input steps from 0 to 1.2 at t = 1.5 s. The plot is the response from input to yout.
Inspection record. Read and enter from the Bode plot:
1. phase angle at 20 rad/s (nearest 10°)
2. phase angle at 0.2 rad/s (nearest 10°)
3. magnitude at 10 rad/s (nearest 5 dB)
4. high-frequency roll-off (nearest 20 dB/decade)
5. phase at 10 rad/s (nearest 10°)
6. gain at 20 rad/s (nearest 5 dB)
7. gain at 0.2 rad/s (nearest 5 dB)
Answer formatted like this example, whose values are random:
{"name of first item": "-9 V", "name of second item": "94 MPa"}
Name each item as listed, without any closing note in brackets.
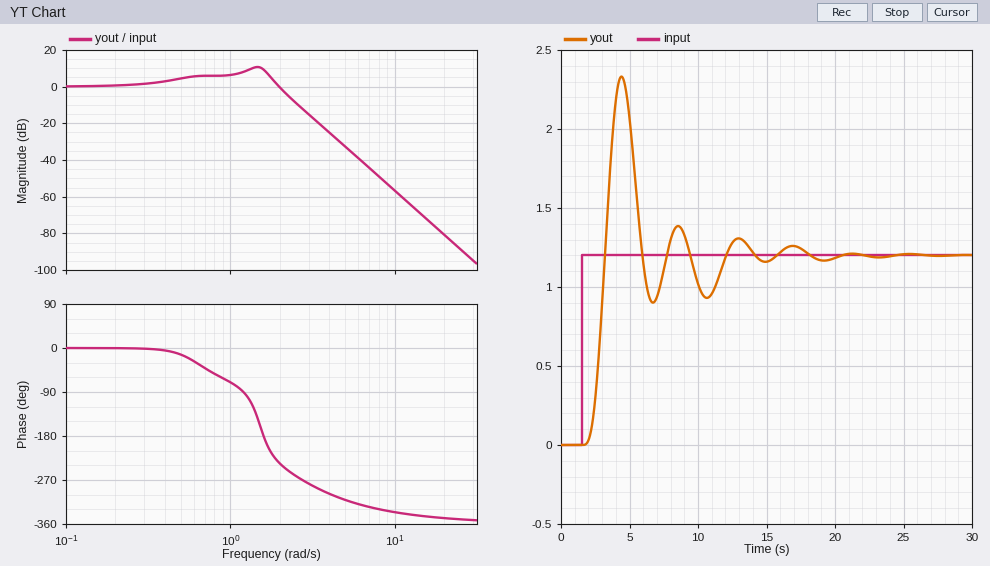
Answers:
{"phase angle at 20 rad/s": "-350°", "phase angle at 0.2 rad/s": "0°", "magnitude at 10 rad/s": "-55 dB", "high-frequency roll-off": "-80 dB/decade", "phase at 10 rad/s": "-340°", "gain at 20 rad/s": "-80 dB", "gain at 0.2 rad/s": "0 dB"}
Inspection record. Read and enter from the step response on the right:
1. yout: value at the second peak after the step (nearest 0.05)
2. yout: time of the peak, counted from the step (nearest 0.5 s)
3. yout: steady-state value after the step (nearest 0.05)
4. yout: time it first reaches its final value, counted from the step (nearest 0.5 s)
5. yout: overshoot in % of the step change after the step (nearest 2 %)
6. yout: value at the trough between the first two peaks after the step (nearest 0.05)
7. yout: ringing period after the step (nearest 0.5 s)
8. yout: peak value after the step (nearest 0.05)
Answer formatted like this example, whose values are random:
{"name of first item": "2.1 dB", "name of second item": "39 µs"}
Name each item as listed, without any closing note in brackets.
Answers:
{"yout: value at the second peak after the step": "1.40", "yout: time of the peak, counted from the step": "3.0 s", "yout: steady-state value after the step": "1.20", "yout: time it first reaches its final value, counted from the step": "1.5 s", "yout: overshoot in % of the step change after the step": "94 %", "yout: value at the trough between the first two peaks after the step": "0.90", "yout: ringing period after the step": "4.0 s", "yout: peak value after the step": "2.35"}
